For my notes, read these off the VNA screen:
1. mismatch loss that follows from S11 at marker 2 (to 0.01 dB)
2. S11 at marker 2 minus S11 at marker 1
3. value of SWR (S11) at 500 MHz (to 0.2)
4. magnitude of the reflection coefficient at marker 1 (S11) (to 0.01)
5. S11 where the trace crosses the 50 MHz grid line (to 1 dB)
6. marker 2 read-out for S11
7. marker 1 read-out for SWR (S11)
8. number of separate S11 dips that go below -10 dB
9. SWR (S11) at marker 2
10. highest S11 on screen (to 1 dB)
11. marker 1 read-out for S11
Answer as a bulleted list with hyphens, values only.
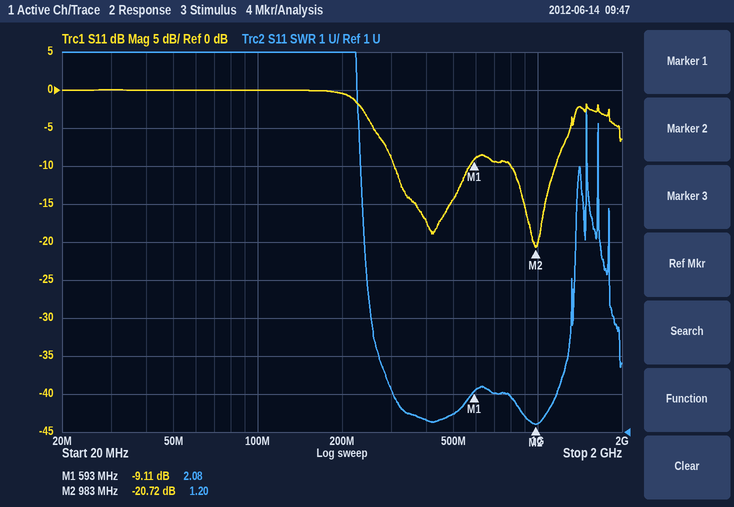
- 0.04 dB
- -11.61 dB
- 1.4
- 0.35
- 0 dB
- -20.72 dB
- 2.08
- 2
- 1.20
- 0 dB
- -9.11 dB
